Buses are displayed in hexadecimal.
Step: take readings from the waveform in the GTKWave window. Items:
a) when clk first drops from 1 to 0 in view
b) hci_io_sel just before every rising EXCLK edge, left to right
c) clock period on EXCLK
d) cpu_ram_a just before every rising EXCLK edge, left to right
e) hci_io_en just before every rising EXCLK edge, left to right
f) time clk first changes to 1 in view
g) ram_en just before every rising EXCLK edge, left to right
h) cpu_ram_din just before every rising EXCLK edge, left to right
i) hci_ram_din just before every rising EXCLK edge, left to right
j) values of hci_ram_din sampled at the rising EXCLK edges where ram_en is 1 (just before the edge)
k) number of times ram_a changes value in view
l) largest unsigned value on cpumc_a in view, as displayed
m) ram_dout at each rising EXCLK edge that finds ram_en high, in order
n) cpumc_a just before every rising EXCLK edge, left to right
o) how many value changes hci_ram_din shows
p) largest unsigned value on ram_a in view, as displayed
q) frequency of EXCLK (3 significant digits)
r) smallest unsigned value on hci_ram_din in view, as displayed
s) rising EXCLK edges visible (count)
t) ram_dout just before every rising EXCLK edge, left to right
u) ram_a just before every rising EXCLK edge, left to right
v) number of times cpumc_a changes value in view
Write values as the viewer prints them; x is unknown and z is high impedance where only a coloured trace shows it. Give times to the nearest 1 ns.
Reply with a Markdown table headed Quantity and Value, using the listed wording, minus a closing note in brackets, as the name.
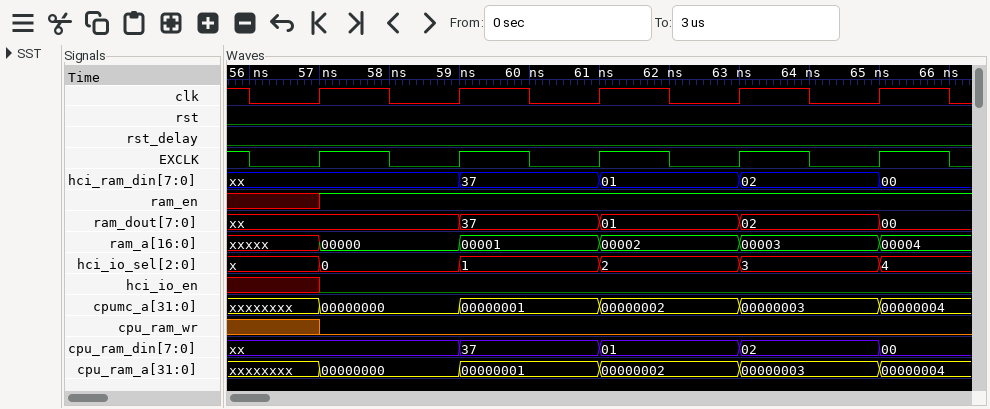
| Quantity | Value |
|---|---|
| when clk first drops from 1 to 0 in view | 56 ns |
| hci_io_sel just before every rising EXCLK edge, left to right | x, 0, 1, 2, 3 |
| clock period on EXCLK | 2 ns |
| cpu_ram_a just before every rising EXCLK edge, left to right | xxxxxxxx, 00000000, 00000001, 00000002, 00000003 |
| hci_io_en just before every rising EXCLK edge, left to right | x 0 0 0 0 |
| time clk first changes to 1 in view | 57 ns |
| ram_en just before every rising EXCLK edge, left to right | x 1 1 1 1 |
| cpu_ram_din just before every rising EXCLK edge, left to right | xx, xx, 37, 01, 02 |
| hci_ram_din just before every rising EXCLK edge, left to right | xx, xx, 37, 01, 02 |
| values of hci_ram_din sampled at the rising EXCLK edges where ram_en is 1 | xx, 37, 01, 02 |
| number of times ram_a changes value in view | 5 |
| largest unsigned value on cpumc_a in view, as displayed | 00000004 |
| ram_dout at each rising EXCLK edge that finds ram_en high, in order | xx, 37, 01, 02 |
| cpumc_a just before every rising EXCLK edge, left to right | xxxxxxxx, 00000000, 00000001, 00000002, 00000003 |
| how many value changes hci_ram_din shows | 4 |
| largest unsigned value on ram_a in view, as displayed | 00004 |
| frequency of EXCLK | 500 MHz |
| smallest unsigned value on hci_ram_din in view, as displayed | 00 |
| rising EXCLK edges visible | 5 |
| ram_dout just before every rising EXCLK edge, left to right | xx, xx, 37, 01, 02 |
| ram_a just before every rising EXCLK edge, left to right | xxxxx, 00000, 00001, 00002, 00003 |
| number of times cpumc_a changes value in view | 5 |
